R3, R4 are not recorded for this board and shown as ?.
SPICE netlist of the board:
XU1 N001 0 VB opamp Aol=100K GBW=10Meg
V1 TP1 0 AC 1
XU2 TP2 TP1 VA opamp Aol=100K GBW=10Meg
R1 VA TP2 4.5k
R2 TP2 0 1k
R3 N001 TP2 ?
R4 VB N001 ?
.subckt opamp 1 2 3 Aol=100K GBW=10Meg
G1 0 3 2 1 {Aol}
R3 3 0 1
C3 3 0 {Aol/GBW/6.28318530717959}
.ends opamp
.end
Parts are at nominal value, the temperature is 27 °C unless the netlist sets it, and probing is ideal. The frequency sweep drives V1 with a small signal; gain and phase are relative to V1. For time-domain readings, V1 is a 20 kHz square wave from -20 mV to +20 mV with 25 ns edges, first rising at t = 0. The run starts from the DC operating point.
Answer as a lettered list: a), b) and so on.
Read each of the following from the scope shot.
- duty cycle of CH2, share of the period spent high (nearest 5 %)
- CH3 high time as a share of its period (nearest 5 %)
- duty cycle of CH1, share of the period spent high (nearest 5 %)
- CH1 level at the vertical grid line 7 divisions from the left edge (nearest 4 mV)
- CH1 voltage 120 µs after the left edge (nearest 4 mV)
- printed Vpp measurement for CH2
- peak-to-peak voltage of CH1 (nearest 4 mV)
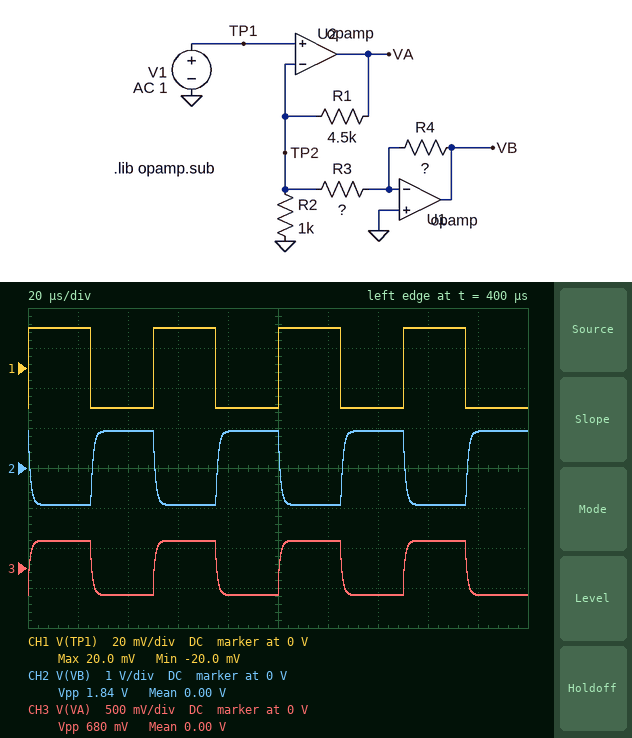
a) 50 %
b) 50 %
c) 50 %
d) -20 mV
e) 20 mV
f) 1.84 V
g) 40 mV
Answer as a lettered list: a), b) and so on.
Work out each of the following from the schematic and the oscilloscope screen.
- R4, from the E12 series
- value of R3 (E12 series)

a) 18 kΩ
b) 390 Ω
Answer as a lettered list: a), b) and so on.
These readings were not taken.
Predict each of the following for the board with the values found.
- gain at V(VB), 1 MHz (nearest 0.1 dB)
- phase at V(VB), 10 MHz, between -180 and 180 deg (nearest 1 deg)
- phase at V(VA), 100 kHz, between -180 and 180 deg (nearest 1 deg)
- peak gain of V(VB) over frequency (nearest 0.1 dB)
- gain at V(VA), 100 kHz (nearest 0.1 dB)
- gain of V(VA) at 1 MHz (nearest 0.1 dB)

a) 16.8 dB
b) 13 deg
c) -24 deg
d) 33.3 dB
e) 23.4 dB
f) 13.7 dB
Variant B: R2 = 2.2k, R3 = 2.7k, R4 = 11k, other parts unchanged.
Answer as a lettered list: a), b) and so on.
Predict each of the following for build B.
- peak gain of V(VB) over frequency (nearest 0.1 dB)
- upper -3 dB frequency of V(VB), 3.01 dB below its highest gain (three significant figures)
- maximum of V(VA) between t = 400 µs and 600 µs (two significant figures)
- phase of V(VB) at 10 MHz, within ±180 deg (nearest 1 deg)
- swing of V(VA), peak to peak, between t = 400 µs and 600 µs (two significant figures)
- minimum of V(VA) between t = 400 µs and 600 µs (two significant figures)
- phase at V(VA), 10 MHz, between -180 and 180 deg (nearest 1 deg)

a) 12.2 dB
b) 1.23 MHz
c) 94 mV
d) 31 deg
e) 190 mV
f) -94 mV
g) -74 deg
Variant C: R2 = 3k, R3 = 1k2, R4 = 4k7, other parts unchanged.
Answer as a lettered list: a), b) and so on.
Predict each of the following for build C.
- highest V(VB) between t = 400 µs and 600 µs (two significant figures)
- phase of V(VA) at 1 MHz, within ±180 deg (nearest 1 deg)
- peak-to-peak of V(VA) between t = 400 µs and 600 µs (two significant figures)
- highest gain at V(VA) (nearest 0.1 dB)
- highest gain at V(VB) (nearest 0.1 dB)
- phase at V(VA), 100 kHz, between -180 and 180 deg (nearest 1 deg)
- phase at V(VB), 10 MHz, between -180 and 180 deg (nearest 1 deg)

a) 78 mV
b) -39 deg
c) 250 mV
d) 15.9 dB
e) 11.9 dB
f) -5 deg
g) 37 deg
